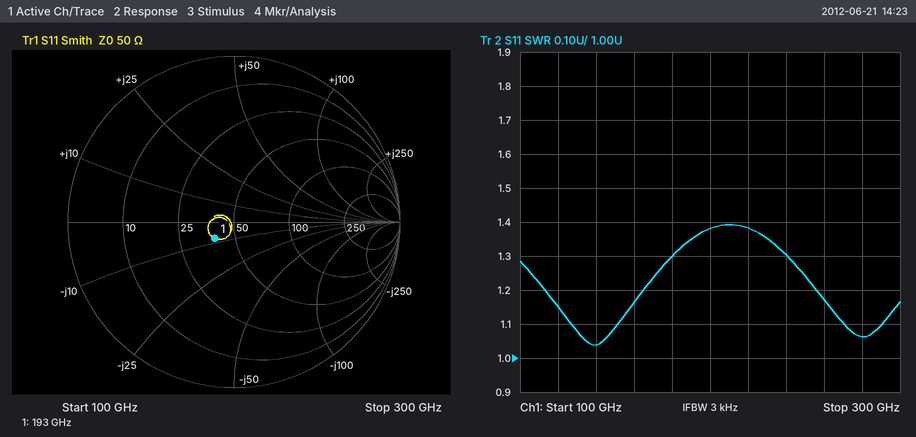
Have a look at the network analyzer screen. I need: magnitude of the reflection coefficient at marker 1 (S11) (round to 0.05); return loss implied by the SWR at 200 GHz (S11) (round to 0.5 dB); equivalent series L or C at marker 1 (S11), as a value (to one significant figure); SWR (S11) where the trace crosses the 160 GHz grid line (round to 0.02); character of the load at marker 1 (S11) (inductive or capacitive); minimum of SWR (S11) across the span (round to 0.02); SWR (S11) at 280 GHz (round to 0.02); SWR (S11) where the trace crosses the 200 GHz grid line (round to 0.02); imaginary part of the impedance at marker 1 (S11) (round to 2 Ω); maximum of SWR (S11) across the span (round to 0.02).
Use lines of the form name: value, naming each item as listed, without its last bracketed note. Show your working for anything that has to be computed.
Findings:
magnitude of the reflection coefficient at marker 1 (S11): 0.15
return loss implied by the SWR at 200 GHz (S11): −20 log10((1.38 − 1)/(1.38 + 1)) ≈ 15.9 dB, so 16.0 dB to the nearest 0.5 dB
equivalent series L or C at marker 1 (S11), as a value: C = 1/(2π × 193 GHz × 8 Ω) ≈ 103 fF, so 100 fF to one significant figure
SWR (S11) where the trace crosses the 160 GHz grid line: 1.16
character of the load at marker 1 (S11): capacitive
minimum of SWR (S11) across the span: 1.04
SWR (S11) at 280 GHz: 1.06
SWR (S11) where the trace crosses the 200 GHz grid line: 1.38
imaginary part of the impedance at marker 1 (S11): -8 Ω
maximum of SWR (S11) across the span: 1.40
